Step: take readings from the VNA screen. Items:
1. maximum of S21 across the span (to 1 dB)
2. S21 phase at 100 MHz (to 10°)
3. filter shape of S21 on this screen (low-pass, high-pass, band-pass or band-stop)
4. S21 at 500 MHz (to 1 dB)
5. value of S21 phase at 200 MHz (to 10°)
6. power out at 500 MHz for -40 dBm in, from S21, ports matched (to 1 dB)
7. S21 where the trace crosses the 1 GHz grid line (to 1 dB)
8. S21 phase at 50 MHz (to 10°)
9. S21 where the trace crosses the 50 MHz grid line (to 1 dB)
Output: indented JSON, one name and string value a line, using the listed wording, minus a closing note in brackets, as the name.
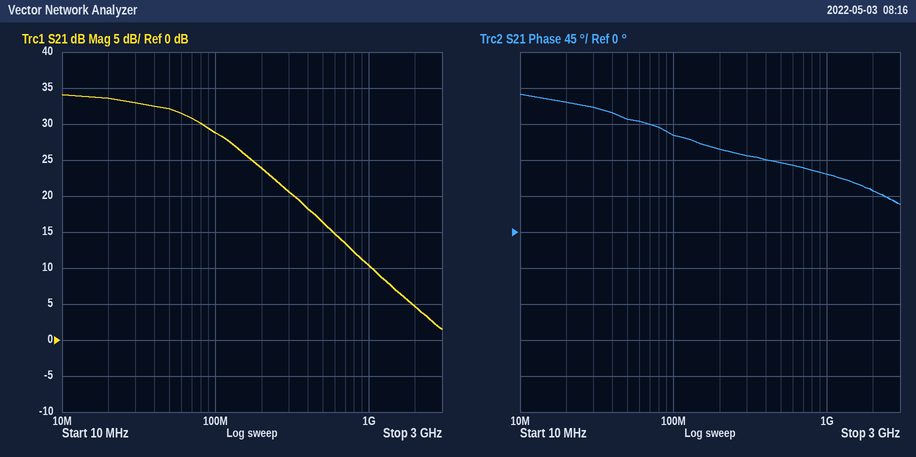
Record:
{
  "maximum of S21 across the span": "34 dB",
  "S21 phase at 100 MHz": "120°",
  "filter shape of S21 on this screen": "low-pass",
  "S21 at 500 MHz": "16 dB",
  "value of S21 phase at 200 MHz": "100°",
  "power out at 500 MHz for -40 dBm in, from S21, ports matched": "-24 dBm",
  "S21 where the trace crosses the 1 GHz grid line": "10 dB",
  "S21 phase at 50 MHz": "140°",
  "S21 where the trace crosses the 50 MHz grid line": "32 dB"
}
